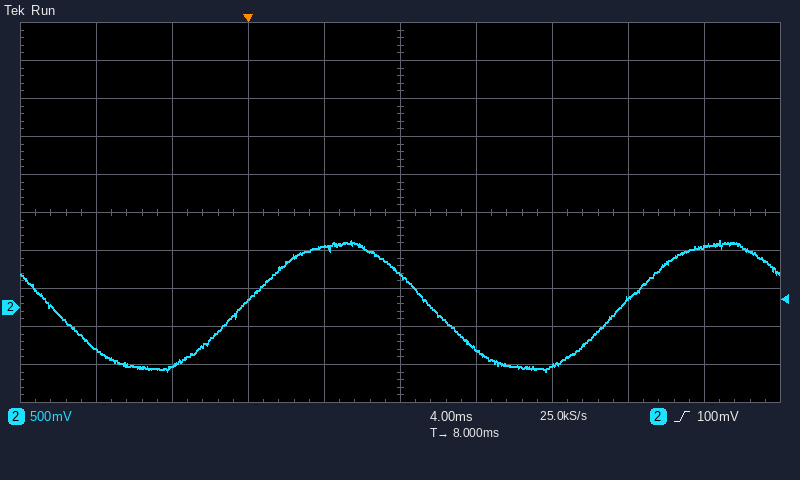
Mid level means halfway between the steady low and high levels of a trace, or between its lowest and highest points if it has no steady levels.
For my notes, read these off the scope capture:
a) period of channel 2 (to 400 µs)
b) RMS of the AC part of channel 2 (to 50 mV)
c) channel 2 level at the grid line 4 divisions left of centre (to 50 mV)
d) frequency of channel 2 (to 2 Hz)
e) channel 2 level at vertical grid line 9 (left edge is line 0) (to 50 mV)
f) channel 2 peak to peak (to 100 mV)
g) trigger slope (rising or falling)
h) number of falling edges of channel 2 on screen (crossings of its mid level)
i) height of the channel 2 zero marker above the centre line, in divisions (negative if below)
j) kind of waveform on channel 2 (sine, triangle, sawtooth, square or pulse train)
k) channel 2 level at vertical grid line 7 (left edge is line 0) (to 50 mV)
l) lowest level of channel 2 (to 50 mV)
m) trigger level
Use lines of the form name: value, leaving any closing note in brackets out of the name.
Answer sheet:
period of channel 2: 20.0 ms
RMS of the AC part of channel 2: 600 mV
channel 2 level at the grid line 4 divisions left of centre: -550 mV
frequency of channel 2: 50 Hz
channel 2 level at vertical grid line 9 (left edge is line 0): 800 mV
channel 2 peak to peak: 1.70 V
trigger slope: rising
number of falling edges of channel 2 on screen: 2
height of the channel 2 zero marker above the centre line, in divisions: -2.5 div
kind of waveform on channel 2: sine
channel 2 level at vertical grid line 7 (left edge is line 0): -750 mV
lowest level of channel 2: -850 mV
trigger level: 100 mV
